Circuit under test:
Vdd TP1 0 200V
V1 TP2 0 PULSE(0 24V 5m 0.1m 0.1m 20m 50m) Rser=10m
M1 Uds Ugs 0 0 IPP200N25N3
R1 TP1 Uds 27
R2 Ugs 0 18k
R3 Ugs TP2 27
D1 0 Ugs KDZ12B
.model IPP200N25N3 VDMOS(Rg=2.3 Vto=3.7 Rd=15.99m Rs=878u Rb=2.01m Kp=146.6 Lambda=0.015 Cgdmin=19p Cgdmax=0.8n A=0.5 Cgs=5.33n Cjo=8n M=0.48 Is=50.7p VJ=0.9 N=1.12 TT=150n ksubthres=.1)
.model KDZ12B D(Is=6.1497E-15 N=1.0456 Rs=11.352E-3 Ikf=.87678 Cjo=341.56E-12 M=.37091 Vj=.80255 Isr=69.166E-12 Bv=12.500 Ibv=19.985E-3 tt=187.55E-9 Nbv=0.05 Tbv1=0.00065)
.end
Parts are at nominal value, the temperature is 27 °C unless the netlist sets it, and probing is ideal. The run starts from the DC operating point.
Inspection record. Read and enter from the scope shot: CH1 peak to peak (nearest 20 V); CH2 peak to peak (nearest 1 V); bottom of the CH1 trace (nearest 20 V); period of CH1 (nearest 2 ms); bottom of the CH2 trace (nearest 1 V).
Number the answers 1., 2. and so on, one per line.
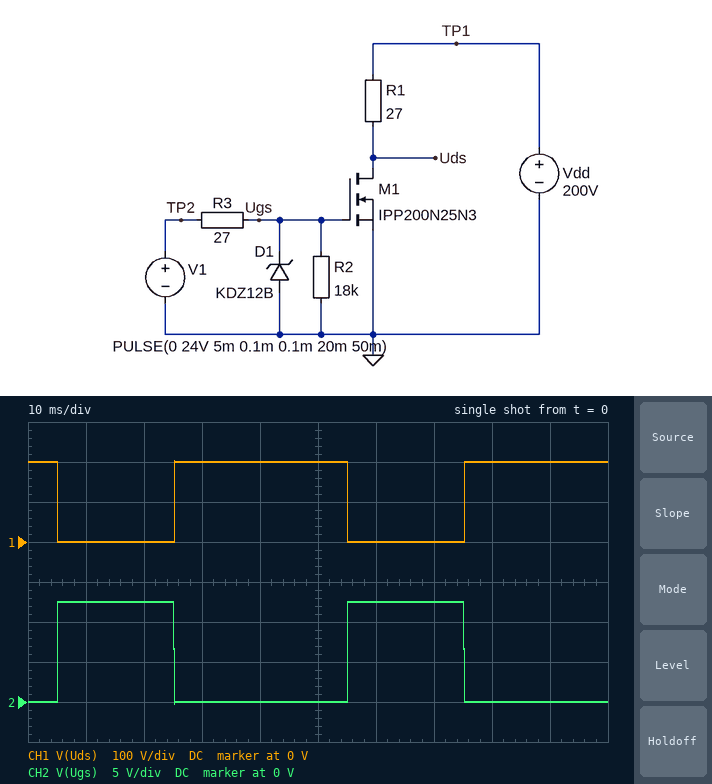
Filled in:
1. 200 V
2. 13 V
3. 0 V
4. 50 ms
5. 0 V
